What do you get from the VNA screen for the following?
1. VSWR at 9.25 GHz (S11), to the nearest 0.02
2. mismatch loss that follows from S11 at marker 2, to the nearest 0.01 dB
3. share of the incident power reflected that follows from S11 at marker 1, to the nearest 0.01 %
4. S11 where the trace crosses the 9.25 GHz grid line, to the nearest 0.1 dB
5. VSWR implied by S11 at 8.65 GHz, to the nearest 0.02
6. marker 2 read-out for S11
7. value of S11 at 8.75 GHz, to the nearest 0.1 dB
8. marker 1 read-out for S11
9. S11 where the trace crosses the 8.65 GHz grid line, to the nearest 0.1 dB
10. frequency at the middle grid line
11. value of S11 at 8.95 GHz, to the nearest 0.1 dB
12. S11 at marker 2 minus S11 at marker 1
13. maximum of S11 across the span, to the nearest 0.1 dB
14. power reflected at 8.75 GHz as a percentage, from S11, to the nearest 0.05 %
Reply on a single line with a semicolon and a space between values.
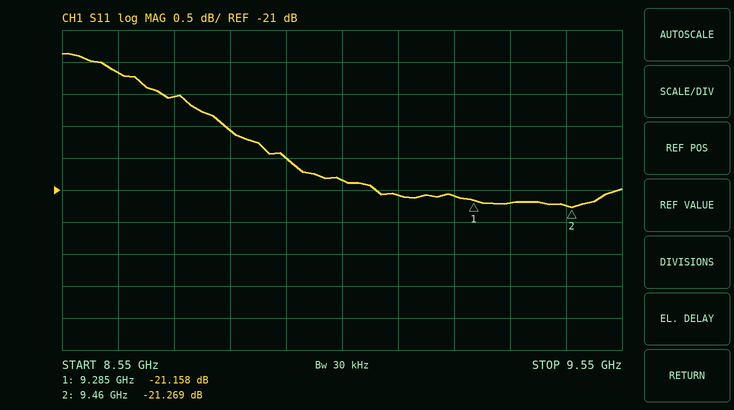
1.20; 0.03 dB; 0.77 %; -21.1 dB; 1.24; -21.269 dB; -19.5 dB; -21.158 dB; -19.2 dB; 9.05 GHz; -20.5 dB; -0.111 dB; -18.9 dB; 1.10 %
